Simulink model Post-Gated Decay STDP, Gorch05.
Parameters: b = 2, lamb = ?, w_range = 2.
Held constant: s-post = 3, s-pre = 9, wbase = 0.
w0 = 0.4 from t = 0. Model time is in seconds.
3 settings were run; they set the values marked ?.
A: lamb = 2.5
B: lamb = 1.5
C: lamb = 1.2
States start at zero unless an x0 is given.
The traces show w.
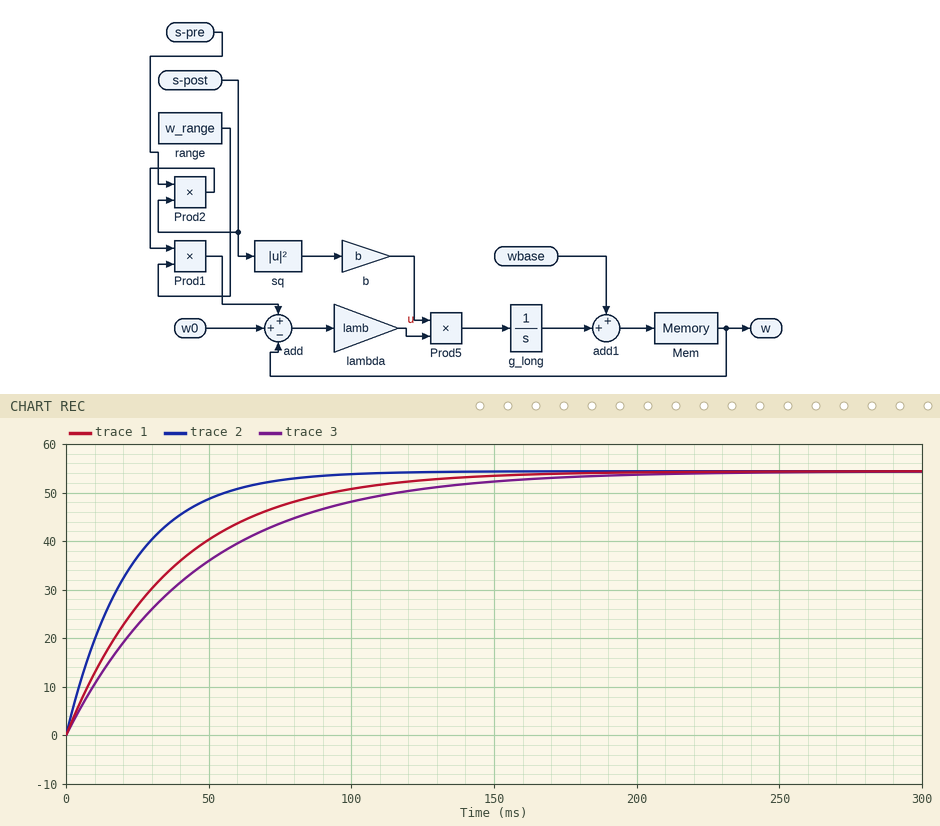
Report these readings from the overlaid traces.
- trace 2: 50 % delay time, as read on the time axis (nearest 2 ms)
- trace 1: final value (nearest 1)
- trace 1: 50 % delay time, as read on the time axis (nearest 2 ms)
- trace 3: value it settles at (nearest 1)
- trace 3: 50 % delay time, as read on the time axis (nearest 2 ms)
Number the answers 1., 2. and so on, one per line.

1. 16 ms
2. 54
3. 26 ms
4. 54
5. 32 ms
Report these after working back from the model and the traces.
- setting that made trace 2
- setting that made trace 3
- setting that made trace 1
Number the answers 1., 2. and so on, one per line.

1. A
2. C
3. B
